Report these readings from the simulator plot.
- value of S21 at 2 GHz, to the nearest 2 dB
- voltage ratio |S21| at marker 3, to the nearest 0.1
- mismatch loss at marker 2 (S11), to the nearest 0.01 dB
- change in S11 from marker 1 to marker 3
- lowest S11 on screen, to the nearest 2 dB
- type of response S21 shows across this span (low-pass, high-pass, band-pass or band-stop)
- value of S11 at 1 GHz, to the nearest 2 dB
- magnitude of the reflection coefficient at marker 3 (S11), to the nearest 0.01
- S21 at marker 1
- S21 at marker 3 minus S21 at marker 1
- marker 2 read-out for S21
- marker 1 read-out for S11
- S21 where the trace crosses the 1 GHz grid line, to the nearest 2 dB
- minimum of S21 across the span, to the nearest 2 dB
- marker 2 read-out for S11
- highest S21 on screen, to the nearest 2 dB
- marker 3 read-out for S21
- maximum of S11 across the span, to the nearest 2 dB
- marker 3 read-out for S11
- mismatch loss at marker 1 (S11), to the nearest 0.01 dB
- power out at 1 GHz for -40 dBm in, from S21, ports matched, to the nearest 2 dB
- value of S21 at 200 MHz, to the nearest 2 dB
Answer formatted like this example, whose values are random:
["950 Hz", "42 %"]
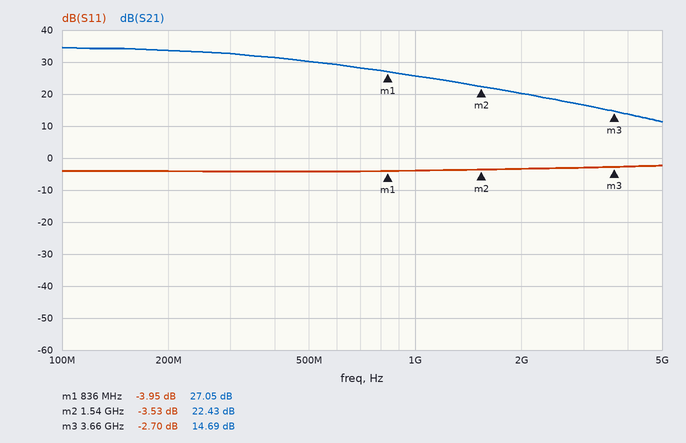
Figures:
["20 dB", "5.4", "2.55 dB", "1.25 dB", "-4 dB", "low-pass", "-4 dB", "0.73", "27.05 dB", "-12.36 dB", "22.43 dB", "-3.95 dB", "26 dB", "12 dB", "-3.53 dB", "34 dB", "14.69 dB", "-2 dB", "-2.70 dB", "2.24 dB", "-14 dBm", "34 dB"]
